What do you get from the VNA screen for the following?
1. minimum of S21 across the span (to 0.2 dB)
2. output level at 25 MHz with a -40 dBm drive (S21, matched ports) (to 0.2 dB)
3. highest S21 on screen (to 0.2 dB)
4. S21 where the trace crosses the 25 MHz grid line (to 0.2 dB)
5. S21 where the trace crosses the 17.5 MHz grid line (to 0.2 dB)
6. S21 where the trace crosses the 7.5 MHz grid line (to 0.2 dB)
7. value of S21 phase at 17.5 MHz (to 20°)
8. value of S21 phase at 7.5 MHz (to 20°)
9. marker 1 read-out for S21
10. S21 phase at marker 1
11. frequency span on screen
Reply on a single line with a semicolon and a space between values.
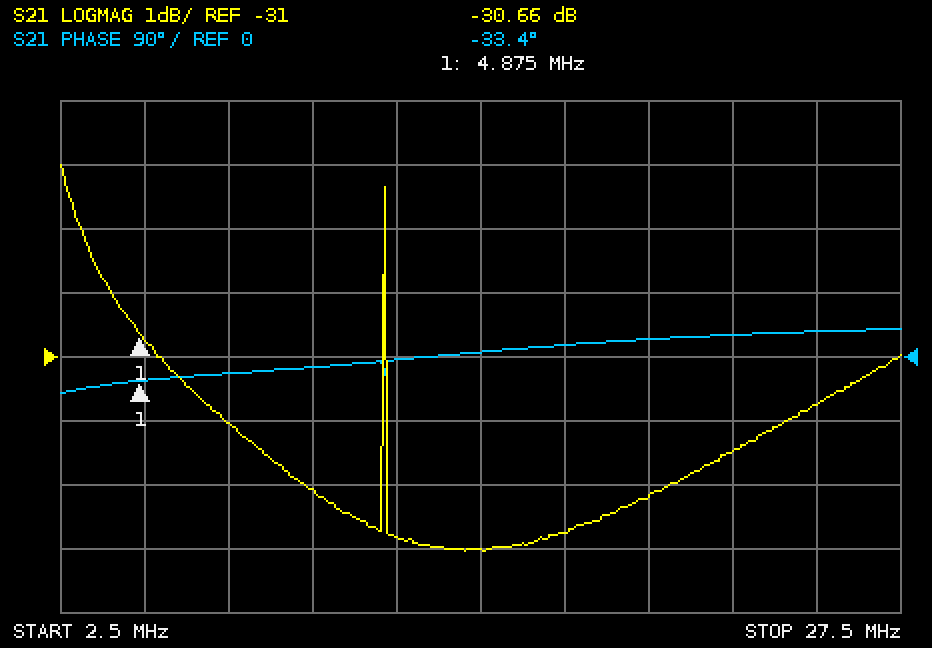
-34.0 dB; -71.8 dBm; -28.0 dB; -31.8 dB; -33.8 dB; -32.0 dB; 20°; -20°; -30.66 dB; -33.4°; 25 MHz
